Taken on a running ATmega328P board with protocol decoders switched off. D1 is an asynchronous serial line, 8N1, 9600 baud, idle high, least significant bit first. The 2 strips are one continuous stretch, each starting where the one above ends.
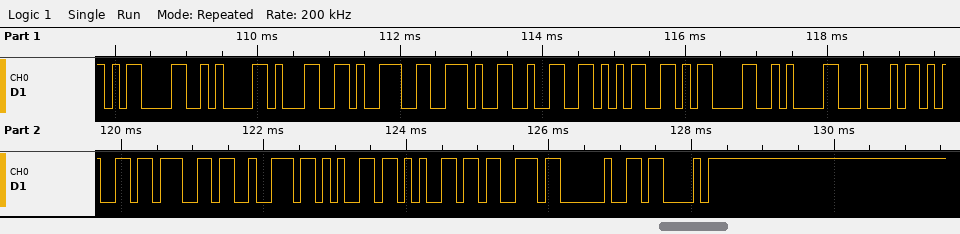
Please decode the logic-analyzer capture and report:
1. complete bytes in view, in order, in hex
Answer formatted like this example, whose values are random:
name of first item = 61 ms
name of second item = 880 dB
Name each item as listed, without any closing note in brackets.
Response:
complete bytes in view, in order, in hex = 0D 0A 31 39 2E 32 35 0D 0A 44 65 67 72 65 65 73 20 43
